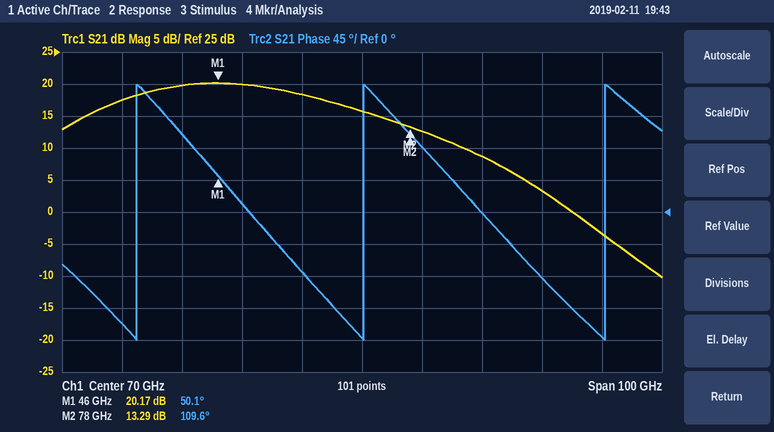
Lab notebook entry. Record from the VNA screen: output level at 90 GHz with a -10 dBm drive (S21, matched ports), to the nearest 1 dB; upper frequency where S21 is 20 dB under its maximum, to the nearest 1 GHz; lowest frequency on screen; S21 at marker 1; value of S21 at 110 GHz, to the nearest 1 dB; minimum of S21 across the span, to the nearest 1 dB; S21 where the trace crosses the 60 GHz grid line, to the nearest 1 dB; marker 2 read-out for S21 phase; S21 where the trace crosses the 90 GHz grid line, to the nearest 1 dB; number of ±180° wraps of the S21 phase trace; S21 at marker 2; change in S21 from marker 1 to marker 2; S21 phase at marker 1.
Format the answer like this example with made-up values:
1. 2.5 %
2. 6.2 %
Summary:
1. -1 dBm
2. 105 GHz
3. 20 GHz
4. 20.17 dB
5. -3 dB
6. -10 dB
7. 18 dB
8. 109.6°
9. 9 dB
10. 3
11. 13.29 dB
12. -6.88 dB
13. 50.1°
